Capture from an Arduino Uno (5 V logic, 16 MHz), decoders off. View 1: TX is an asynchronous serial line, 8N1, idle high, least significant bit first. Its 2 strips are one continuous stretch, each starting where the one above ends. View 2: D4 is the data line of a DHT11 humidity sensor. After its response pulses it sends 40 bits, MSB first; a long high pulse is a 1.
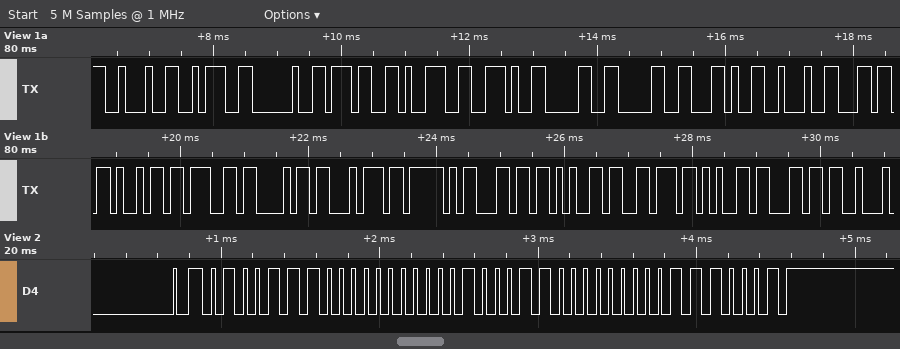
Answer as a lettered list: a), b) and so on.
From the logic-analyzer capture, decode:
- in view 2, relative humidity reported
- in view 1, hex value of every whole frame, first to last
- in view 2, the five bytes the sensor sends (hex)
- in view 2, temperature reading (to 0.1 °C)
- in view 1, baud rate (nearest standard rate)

a) 78 %
b) 22 3A 20 37 39 2E 30 30 2C 22 6C 69 67 68 74 5F 6C 65 76 65 6C
c) 4E 00 23 00 71
d) 35.0 °C
e) 9600 baud
